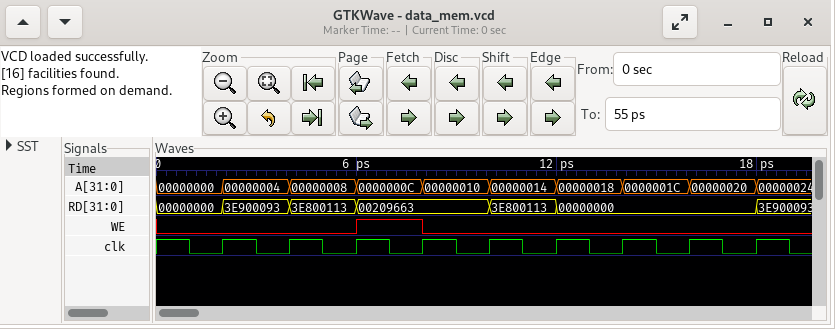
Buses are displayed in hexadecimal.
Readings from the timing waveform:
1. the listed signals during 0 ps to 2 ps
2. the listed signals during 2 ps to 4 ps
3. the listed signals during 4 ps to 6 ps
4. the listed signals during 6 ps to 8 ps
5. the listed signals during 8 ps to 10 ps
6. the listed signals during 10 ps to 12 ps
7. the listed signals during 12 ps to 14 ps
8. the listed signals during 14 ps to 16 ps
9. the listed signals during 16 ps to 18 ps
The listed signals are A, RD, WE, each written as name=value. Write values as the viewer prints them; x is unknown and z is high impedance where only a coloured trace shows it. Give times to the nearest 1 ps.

A=00000000, RD=00000000, WE=0
A=00000004, RD=3E900093, WE=0
A=00000008, RD=3E800113, WE=0
A=0000000C, RD=00209663, WE=1
A=00000010, RD=00209663, WE=0
A=00000014, RD=3E800113, WE=0
A=00000018, RD=00000000, WE=0
A=0000001C, RD=00000000, WE=0
A=00000020, RD=00000000, WE=0
